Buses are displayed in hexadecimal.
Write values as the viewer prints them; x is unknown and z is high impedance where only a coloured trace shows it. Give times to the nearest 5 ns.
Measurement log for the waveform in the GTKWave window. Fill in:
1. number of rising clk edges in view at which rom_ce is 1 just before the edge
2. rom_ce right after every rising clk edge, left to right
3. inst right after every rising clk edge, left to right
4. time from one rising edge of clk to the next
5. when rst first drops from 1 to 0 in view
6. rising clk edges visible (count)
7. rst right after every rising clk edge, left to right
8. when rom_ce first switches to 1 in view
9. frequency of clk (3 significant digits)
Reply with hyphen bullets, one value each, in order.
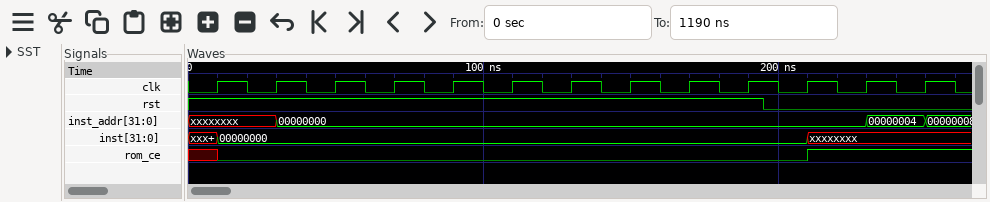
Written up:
- 2
- 0 0 0 0 0 0 0 0 0 0 1 1 1
- 00000000, 00000000, 00000000, 00000000, 00000000, 00000000, 00000000, 00000000, 00000000, 00000000, xxxxxxxx, xxxxxxxx, xxxxxxxx
- 20 ns
- 195 ns
- 13
- 1 1 1 1 1 1 1 1 1 1 0 0 0
- 210 ns
- 50.0 MHz
